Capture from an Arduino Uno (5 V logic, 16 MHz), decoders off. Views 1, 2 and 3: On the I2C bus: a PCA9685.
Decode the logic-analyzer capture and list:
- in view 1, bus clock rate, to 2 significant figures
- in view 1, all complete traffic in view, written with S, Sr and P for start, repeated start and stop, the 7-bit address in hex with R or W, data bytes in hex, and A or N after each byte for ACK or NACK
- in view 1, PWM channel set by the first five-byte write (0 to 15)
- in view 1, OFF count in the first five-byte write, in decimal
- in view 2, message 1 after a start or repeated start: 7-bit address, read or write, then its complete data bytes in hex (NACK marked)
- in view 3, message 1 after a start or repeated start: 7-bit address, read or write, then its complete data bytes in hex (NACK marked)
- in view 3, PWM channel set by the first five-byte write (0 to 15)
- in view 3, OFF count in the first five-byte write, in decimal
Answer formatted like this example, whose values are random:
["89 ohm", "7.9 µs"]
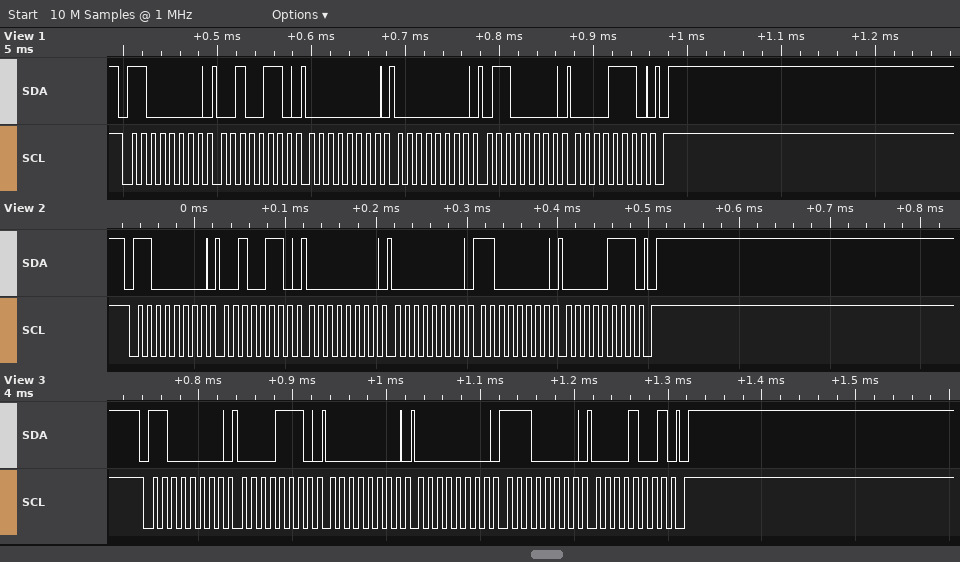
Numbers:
["100 kHz", "S 60W A 26 A 00 A 00 A 60 A 0E A P", "8", "3680", "0x60 write: 26 00 00 C0 07", "0x60 write: 0E 00 00 E0 09", "2", "2528"]
